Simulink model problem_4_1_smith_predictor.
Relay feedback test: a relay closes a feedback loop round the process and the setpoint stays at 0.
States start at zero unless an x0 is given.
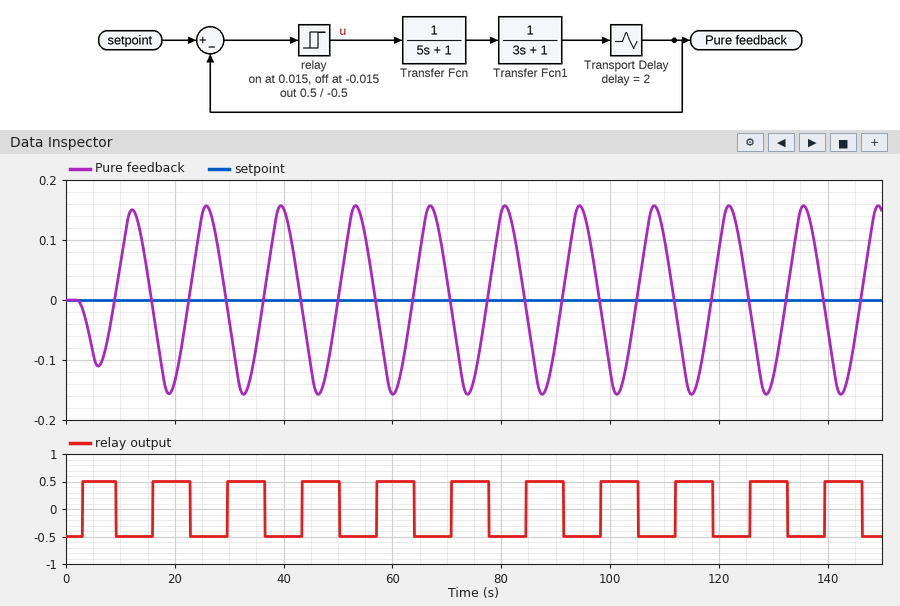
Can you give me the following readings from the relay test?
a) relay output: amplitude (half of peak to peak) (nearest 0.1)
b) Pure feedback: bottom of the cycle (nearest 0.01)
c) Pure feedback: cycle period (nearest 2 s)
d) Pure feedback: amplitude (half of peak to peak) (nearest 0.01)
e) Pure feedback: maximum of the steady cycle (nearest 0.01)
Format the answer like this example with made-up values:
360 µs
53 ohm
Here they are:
0.5
-0.16
14 s
0.16
0.16
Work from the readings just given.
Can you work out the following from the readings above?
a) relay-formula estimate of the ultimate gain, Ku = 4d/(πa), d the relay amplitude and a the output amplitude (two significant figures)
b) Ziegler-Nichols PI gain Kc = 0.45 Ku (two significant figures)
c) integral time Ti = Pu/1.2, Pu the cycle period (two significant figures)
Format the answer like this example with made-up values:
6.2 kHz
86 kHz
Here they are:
4.0
1.8
12 s
